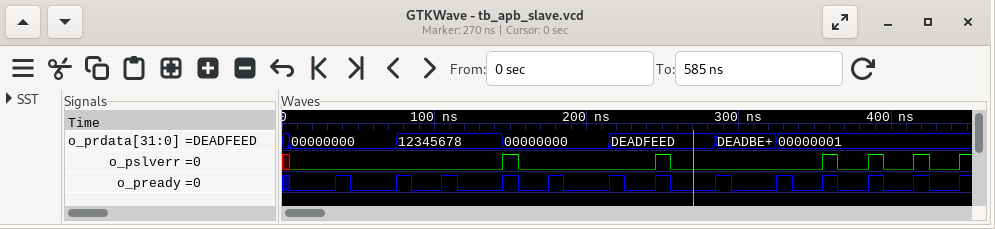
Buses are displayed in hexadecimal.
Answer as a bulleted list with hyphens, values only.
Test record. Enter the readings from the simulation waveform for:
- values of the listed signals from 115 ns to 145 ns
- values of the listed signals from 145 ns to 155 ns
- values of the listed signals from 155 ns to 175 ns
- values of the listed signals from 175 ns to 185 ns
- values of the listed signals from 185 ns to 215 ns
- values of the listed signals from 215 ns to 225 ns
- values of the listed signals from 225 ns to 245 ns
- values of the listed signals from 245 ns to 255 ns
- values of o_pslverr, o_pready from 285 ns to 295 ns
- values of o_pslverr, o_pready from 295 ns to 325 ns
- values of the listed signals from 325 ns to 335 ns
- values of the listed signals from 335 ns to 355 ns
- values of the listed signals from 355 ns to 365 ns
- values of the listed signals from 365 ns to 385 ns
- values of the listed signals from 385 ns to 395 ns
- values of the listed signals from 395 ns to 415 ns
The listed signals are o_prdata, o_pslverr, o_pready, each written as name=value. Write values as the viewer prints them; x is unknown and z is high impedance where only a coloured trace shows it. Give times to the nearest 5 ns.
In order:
- o_prdata=12345678, o_pslverr=0, o_pready=0
- o_prdata=00000000, o_pslverr=1, o_pready=1
- o_prdata=00000000, o_pslverr=0, o_pready=0
- o_prdata=00000000, o_pslverr=0, o_pready=1
- o_prdata=00000000, o_pslverr=0, o_pready=0
- o_prdata=DEADFEED, o_pslverr=0, o_pready=1
- o_prdata=DEADFEED, o_pslverr=0, o_pready=0
- o_prdata=DEADFEED, o_pslverr=1, o_pready=1
- o_pslverr=0, o_pready=1
- o_pslverr=0, o_pready=0
- o_prdata=00000001, o_pslverr=0, o_pready=1
- o_prdata=00000001, o_pslverr=0, o_pready=0
- o_prdata=00000001, o_pslverr=1, o_pready=1
- o_prdata=00000001, o_pslverr=0, o_pready=0
- o_prdata=00000001, o_pslverr=1, o_pready=1
- o_prdata=00000001, o_pslverr=0, o_pready=0
